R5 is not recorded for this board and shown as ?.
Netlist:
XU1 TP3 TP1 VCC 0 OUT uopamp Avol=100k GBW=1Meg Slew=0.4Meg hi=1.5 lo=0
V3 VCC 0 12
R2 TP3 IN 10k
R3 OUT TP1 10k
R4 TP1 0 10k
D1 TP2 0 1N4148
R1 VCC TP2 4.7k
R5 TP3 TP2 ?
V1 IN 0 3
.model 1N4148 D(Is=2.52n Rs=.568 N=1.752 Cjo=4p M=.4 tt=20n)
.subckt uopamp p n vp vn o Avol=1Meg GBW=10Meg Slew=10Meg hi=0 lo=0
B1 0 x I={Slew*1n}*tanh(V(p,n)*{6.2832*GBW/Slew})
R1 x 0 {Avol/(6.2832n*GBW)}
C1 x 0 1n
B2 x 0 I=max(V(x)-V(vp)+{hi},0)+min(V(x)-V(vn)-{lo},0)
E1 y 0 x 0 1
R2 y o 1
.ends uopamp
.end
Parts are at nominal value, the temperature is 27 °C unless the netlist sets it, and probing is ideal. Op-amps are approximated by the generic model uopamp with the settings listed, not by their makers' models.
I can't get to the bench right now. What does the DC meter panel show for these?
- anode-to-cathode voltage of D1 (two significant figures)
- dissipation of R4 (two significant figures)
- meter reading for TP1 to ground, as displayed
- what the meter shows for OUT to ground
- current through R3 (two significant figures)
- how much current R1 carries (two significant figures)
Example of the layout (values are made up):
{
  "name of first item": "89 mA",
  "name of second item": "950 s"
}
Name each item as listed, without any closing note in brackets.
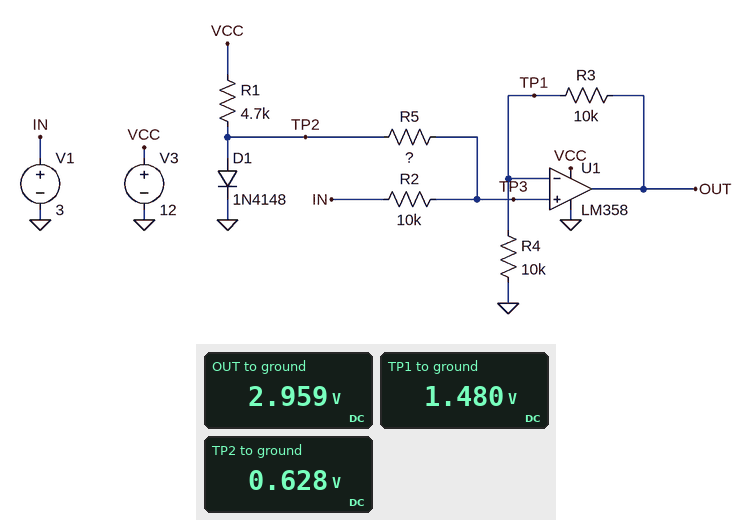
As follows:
{
  "anode-to-cathode voltage of D1": "630 mV",
  "dissipation of R4": "220 µW",
  "meter reading for TP1 to ground, as displayed": "1.480 V",
  "what the meter shows for OUT to ground": "2.959 V",
  "current through R3": "150 µA",
  "how much current R1 carries": "2.4 mA"
}
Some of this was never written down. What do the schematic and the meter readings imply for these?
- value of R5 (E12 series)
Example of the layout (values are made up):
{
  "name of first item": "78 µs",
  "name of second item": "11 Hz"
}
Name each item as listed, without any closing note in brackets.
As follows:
{
  "value of R5": "5.6 kΩ"
}
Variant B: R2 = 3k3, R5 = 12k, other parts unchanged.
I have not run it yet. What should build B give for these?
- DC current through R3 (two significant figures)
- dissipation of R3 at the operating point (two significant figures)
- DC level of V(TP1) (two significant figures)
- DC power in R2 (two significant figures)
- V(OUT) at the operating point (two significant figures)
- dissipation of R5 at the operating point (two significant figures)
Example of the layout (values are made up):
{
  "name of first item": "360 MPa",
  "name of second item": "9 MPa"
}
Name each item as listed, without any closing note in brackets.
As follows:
{
  "DC current through R3": "250 µA",
  "dissipation of R3 at the operating point": "620 µW",
  "DC level of V(TP1)": "2.5 V",
  "DC power in R2": "79 µW",
  "V(OUT) at the operating point": "5.0 V",
  "dissipation of R5 at the operating point": "290 µW"
}
